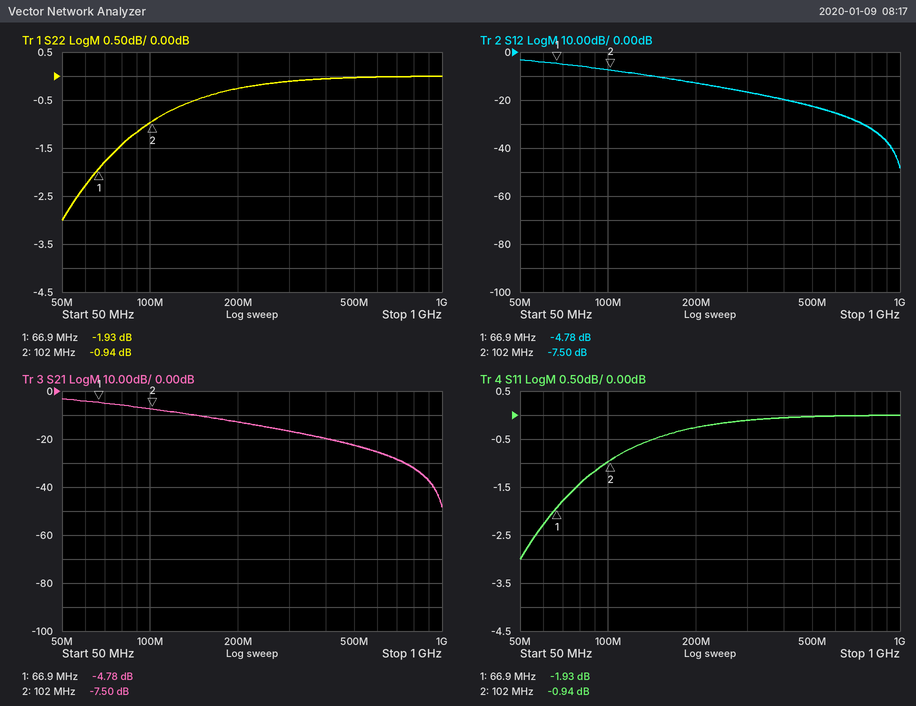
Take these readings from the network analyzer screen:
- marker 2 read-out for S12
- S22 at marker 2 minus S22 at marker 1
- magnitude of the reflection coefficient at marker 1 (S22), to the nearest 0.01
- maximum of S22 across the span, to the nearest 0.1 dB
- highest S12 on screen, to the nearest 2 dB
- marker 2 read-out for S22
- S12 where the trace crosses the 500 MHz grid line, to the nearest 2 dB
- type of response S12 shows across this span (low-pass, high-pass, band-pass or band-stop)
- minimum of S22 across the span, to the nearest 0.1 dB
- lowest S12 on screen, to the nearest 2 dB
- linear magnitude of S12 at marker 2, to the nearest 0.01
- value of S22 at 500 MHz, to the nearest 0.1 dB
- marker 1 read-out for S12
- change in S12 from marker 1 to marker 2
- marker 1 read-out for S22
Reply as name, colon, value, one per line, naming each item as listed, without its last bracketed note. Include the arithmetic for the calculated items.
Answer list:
marker 2 read-out for S12: -7.50 dB
S22 at marker 2 minus S22 at marker 1: -0.94 − (-1.93) = 0.99 dB
magnitude of the reflection coefficient at marker 1 (S22), to the nearest 0.01: 10^(-1.93/20) ≈ 0.80
maximum of S22 across the span, to the nearest 0.1 dB: 0.0 dB
highest S12 on screen, to the nearest 2 dB: -4 dB
marker 2 read-out for S22: -0.94 dB
S12 where the trace crosses the 500 MHz grid line, to the nearest 2 dB: -22 dB
type of response S12 shows across this span: low-pass
minimum of S22 across the span, to the nearest 0.1 dB: -3.0 dB
lowest S12 on screen, to the nearest 2 dB: -48 dB
linear magnitude of S12 at marker 2, to the nearest 0.01: 10^(-7.5/20) ≈ 0.42
value of S22 at 500 MHz, to the nearest 0.1 dB: 0.0 dB
marker 1 read-out for S12: -4.78 dB
change in S12 from marker 1 to marker 2: -7.5 − (-4.78) = -2.72 dB
marker 1 read-out for S22: -1.93 dB
